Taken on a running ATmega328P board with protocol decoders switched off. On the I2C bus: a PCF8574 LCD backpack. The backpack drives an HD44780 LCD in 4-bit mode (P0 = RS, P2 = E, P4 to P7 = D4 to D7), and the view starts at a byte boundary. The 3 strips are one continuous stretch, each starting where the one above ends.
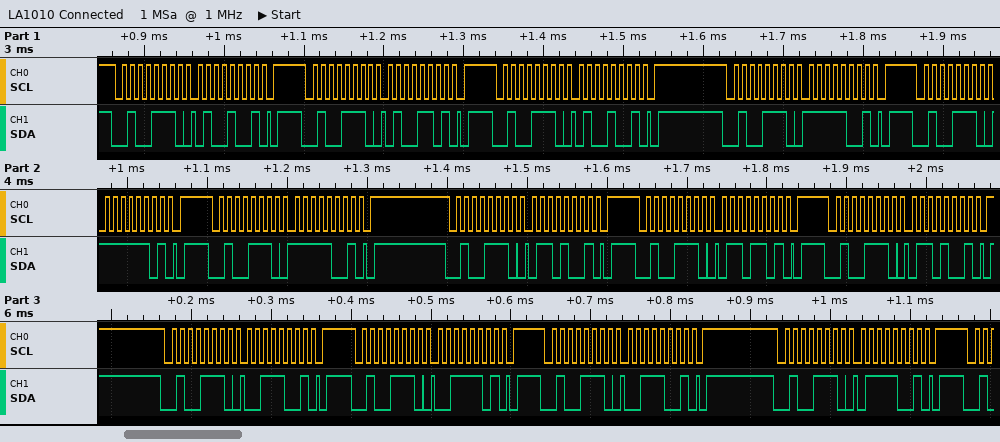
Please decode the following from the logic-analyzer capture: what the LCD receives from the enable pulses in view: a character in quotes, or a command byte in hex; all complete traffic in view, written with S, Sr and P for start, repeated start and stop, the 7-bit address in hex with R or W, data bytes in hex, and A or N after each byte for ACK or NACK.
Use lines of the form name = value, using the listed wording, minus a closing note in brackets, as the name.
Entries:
what the LCD receives from the enable pulses in view: a character in quotes, or a command byte in hex = 'O' 'c'
all complete traffic in view, written with S, Sr and P for start, repeated start and stop, the 7-bit address in hex with R or W, data bytes in hex, and A or N after each byte for ACK or NACK = S 27W A 49 A P S 27W A 4D A P S 27W A 49 A P S 27W A F9 A P S 27W A FD A P S 27W A F9 A P S 27W A 69 A P S 27W A 6D A P S 27W A 69 A P S 27W A 39 A P S 27W A 3D A P S 27W A 39 A P S 27W A 79 A P
